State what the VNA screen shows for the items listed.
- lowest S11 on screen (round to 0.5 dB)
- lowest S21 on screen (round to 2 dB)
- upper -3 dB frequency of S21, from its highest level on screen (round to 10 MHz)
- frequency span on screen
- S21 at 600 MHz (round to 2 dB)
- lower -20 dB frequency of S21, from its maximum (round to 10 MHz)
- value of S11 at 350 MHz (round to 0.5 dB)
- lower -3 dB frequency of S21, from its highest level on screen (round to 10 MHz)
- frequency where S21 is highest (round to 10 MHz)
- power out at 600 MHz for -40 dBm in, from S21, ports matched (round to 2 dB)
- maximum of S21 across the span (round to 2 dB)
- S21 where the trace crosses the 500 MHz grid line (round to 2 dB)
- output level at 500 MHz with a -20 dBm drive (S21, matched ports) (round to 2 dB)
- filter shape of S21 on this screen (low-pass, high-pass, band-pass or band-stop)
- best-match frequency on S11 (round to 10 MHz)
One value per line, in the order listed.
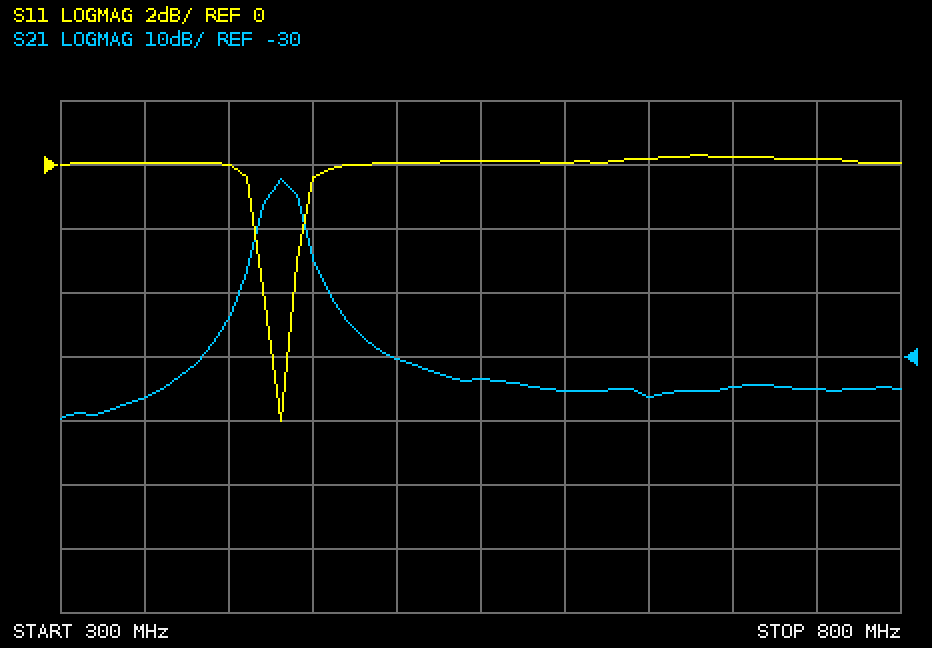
-8.0 dB
-40 dB
440 MHz
500 MHz
-36 dB
400 MHz
0.0 dB
420 MHz
430 MHz
-76 dBm
-2 dB
-30 dB
-50 dBm
band-pass
430 MHz
